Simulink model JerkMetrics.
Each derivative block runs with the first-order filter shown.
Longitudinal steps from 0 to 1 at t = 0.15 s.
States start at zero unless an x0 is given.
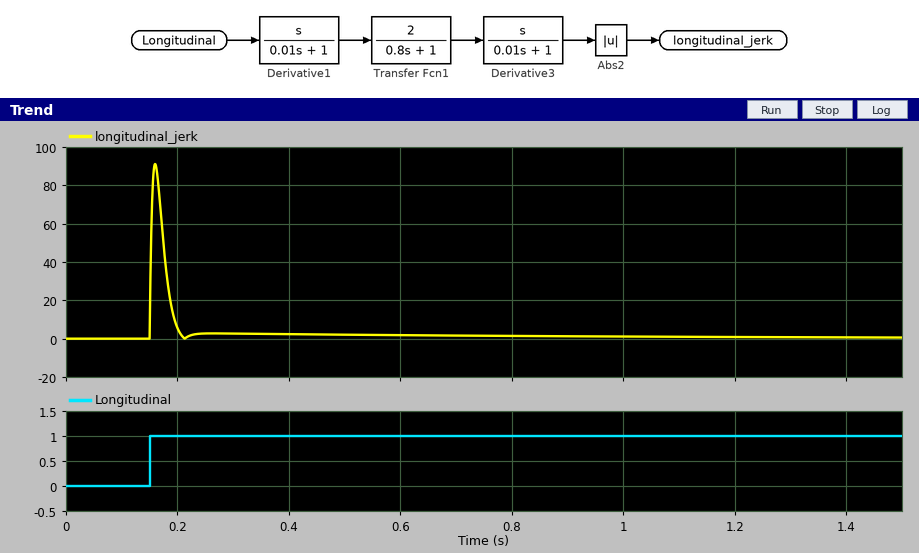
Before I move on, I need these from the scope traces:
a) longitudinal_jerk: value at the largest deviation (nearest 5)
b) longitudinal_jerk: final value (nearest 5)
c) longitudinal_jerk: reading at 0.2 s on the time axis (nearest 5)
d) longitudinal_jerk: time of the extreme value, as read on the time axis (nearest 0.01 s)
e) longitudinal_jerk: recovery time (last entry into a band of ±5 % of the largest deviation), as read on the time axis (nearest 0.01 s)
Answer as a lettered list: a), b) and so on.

a) 90
b) 0
c) 5
d) 0.16 s
e) 0.20 s
